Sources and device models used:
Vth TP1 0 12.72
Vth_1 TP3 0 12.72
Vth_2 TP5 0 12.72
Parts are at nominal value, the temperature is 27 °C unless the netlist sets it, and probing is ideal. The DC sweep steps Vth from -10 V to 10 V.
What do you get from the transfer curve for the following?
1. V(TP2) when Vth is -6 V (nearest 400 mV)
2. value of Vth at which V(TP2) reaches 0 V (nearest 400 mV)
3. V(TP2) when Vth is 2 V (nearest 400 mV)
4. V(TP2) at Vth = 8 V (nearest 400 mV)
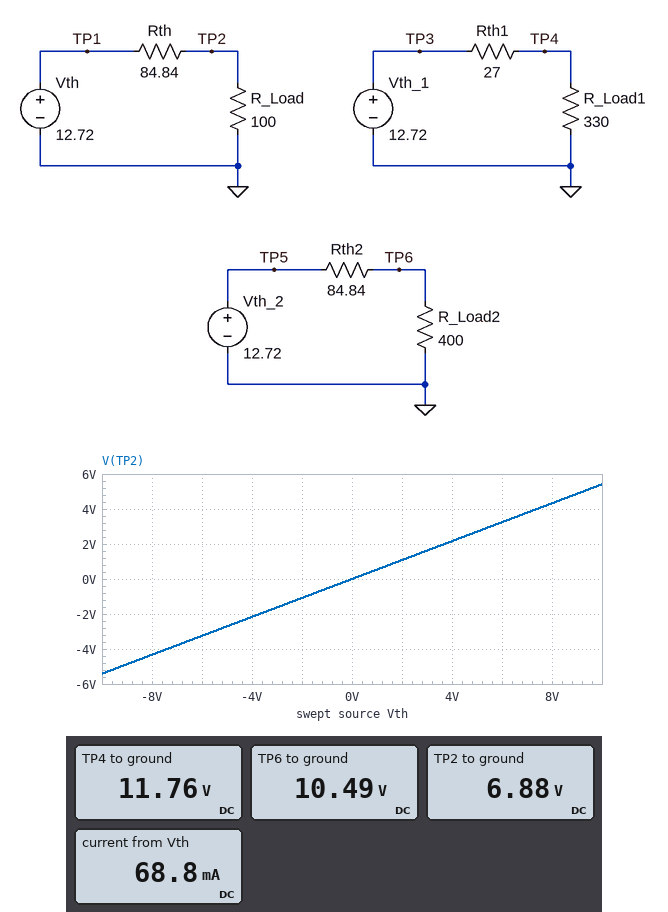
-3.2 V
0 V
1.2 V
4.4 V
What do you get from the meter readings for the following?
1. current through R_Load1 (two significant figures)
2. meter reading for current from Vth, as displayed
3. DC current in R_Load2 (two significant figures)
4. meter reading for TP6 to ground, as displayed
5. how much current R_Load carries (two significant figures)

36 mA
68.8 mA
26 mA
10.49 V
69 mA
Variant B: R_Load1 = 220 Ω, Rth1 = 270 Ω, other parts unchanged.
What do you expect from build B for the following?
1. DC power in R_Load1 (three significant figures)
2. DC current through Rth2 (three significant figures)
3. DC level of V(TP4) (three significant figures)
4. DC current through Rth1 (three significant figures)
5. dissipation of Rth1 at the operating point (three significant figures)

148 mW
26.2 mA
5.71 V
26.0 mA
182 mW
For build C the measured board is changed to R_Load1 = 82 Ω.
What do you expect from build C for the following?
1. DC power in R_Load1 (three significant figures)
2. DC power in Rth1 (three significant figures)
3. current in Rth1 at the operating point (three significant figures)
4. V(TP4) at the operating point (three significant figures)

1.12 W
368 mW
117 mA
9.57 V
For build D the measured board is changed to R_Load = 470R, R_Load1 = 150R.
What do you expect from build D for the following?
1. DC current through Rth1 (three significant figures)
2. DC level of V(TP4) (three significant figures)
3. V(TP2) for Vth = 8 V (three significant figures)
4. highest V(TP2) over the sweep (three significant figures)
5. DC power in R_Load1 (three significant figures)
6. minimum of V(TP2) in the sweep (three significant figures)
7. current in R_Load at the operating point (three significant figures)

71.9 mA
10.8 V
6.78 V
8.47 V
775 mW
-8.47 V
22.9 mA
